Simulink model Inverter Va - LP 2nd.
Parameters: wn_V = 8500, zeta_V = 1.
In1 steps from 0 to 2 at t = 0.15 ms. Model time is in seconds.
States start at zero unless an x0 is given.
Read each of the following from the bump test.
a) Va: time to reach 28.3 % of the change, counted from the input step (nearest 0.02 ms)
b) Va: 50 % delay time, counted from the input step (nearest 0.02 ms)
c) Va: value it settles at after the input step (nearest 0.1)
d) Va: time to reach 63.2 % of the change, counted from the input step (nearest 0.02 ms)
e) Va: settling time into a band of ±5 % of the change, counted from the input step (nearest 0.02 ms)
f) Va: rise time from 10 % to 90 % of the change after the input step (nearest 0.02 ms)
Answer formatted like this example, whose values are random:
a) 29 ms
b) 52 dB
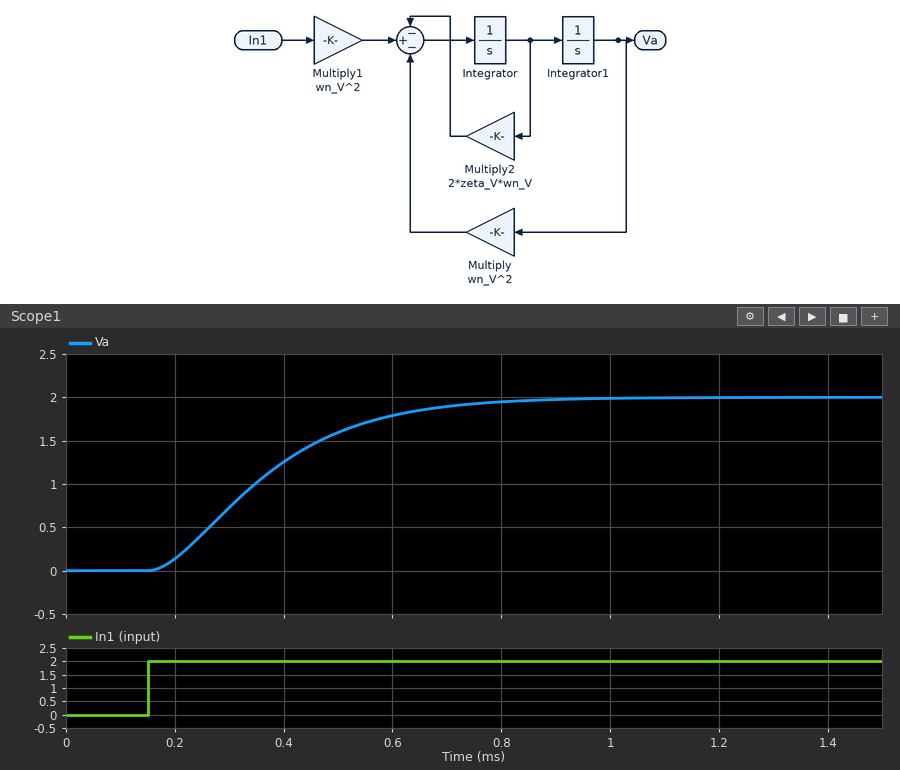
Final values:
a) 0.12 ms
b) 0.20 ms
c) 2.0
d) 0.26 ms
e) 0.56 ms
f) 0.40 ms
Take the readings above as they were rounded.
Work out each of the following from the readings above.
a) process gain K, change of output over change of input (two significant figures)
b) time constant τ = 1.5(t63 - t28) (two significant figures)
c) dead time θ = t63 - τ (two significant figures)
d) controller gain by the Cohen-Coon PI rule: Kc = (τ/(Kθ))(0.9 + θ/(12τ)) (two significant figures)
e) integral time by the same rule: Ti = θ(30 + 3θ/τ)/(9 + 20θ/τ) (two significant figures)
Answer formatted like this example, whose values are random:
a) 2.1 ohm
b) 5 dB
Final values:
a) 1.0
b) 0.21 ms
c) 0.050 ms
d) 3.9
e) 0.11 ms
